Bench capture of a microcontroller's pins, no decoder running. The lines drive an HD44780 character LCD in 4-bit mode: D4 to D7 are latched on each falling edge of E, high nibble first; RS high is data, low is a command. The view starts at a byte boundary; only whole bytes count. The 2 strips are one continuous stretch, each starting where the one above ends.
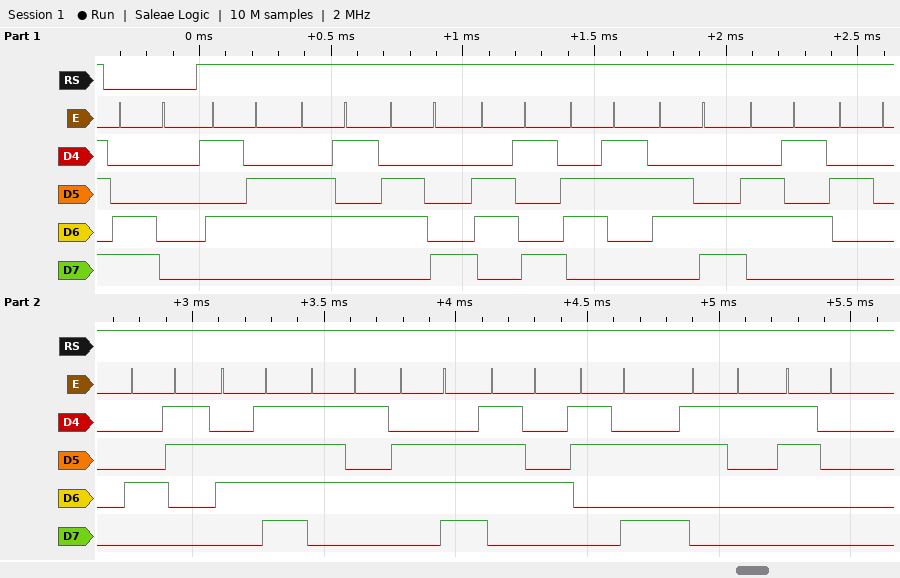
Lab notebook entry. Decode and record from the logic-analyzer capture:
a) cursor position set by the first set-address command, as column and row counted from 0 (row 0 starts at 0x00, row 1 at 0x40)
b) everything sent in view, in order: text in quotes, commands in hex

column 0, row 1
0xC0 "Vehicle Count:10"
